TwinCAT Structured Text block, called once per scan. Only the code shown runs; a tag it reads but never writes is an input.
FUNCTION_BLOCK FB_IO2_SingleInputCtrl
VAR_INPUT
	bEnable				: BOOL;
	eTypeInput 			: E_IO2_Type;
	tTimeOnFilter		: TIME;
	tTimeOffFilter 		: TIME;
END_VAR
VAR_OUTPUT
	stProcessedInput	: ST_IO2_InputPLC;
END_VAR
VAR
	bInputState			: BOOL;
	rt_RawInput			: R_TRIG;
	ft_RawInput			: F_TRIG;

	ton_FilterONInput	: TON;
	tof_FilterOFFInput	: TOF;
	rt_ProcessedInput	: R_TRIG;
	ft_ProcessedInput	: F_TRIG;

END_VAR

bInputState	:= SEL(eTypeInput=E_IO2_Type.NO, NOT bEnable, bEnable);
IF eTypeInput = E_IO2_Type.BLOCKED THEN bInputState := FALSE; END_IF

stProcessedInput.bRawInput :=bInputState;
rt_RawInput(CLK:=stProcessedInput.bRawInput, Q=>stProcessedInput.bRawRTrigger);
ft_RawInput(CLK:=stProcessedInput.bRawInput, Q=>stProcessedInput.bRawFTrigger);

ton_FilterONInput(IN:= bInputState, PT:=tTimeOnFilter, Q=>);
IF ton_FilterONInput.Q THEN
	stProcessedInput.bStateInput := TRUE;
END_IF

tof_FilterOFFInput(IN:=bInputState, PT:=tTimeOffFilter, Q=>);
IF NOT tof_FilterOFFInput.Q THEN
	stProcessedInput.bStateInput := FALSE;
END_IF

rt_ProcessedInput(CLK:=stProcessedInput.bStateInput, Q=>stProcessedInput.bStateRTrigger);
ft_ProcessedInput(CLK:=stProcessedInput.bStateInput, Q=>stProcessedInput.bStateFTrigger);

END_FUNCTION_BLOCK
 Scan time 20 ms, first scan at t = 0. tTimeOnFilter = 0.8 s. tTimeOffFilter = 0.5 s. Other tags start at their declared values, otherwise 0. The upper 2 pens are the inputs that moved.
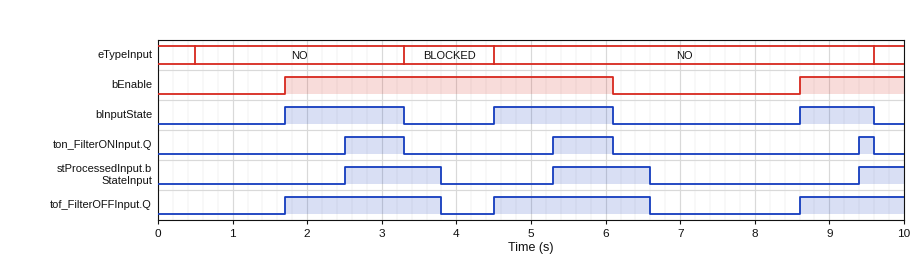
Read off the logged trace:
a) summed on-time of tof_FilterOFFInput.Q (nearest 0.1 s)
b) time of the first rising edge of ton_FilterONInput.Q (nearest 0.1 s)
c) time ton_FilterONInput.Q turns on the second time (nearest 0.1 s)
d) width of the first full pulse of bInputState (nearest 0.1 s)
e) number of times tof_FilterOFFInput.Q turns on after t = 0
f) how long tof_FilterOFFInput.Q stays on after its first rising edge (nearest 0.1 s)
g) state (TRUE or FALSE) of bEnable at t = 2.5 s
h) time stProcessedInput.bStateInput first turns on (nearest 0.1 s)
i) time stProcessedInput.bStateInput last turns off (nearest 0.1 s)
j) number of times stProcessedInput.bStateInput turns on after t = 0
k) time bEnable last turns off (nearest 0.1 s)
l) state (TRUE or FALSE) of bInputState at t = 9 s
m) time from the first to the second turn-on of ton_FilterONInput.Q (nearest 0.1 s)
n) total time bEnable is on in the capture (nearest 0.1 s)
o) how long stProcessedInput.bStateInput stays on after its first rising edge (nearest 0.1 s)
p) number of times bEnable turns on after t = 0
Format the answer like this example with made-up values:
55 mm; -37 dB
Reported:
5.6 s; 2.5 s; 5.3 s; 1.6 s; 3; 2.1 s; TRUE; 2.5 s; 6.6 s; 3; 6.1 s; TRUE; 2.8 s; 5.8 s; 1.3 s; 2
